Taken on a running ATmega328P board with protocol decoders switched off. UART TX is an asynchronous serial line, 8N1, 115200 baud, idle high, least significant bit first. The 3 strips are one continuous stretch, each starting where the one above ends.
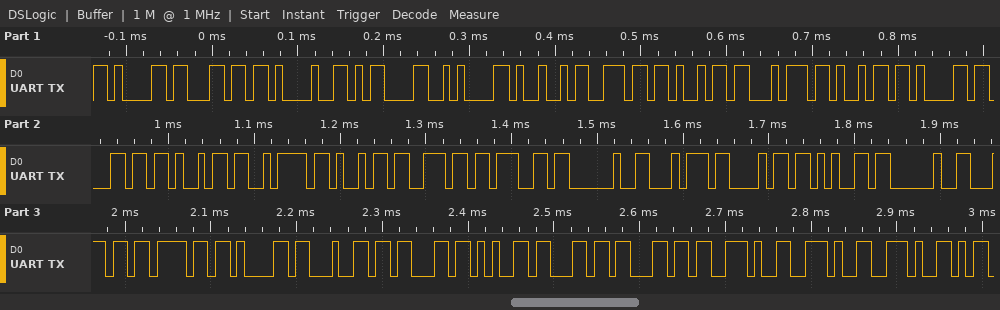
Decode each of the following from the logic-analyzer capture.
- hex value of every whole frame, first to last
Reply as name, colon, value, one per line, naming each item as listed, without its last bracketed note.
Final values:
hex value of every whole frame, first to last: 61 6C 21 0D 0A 49 6E 69 74 69 61 6C 69 7A 69 6E 67 20 74 68 65 20 6C 6F 61 64 63 65 6C 6C 2E 2E 2E
